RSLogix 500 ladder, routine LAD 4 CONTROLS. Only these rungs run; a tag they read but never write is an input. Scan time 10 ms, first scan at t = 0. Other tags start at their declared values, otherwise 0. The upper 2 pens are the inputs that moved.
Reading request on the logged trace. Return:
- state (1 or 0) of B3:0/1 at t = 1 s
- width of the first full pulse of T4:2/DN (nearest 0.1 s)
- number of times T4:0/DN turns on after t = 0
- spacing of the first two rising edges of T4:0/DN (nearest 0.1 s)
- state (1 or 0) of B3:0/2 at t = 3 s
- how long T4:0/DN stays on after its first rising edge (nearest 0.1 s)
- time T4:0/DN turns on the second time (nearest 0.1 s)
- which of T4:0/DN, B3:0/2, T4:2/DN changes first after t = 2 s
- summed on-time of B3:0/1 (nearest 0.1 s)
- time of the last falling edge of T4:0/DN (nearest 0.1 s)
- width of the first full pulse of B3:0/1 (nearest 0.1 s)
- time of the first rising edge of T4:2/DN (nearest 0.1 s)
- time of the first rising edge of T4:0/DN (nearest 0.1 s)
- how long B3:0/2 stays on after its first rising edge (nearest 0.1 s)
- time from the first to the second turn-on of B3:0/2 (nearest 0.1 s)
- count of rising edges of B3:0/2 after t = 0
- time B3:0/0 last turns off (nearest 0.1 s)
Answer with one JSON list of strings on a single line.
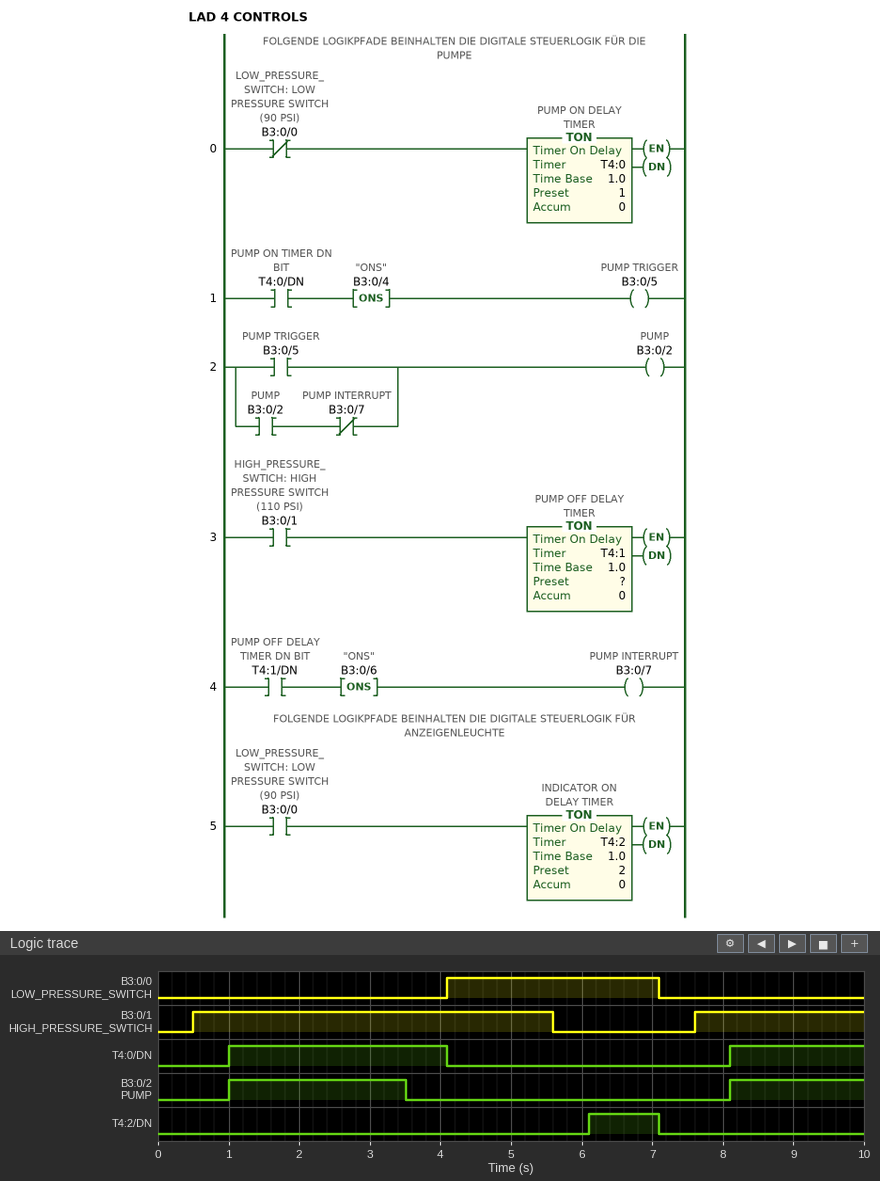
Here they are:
["1", "1.0 s", "2", "7.1 s", "1", "3.1 s", "8.1 s", "B3:0/2", "7.5 s", "4.1 s", "5.1 s", "6.1 s", "1.0 s", "2.5 s", "7.1 s", "2", "7.1 s"]
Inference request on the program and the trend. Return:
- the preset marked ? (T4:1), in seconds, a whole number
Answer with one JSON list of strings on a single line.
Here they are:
["3 s"]
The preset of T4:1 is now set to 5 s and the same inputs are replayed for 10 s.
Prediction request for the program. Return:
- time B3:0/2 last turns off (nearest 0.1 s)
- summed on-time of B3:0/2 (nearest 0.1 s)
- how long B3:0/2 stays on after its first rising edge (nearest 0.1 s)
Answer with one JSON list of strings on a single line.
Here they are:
["5.5 s", "6.4 s", "4.5 s"]
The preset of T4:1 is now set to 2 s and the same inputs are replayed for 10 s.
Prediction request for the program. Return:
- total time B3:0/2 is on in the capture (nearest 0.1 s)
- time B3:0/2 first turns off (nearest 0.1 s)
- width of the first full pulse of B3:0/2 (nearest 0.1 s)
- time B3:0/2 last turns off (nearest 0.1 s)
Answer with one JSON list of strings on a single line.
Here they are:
["3.0 s", "2.5 s", "1.5 s", "9.6 s"]
